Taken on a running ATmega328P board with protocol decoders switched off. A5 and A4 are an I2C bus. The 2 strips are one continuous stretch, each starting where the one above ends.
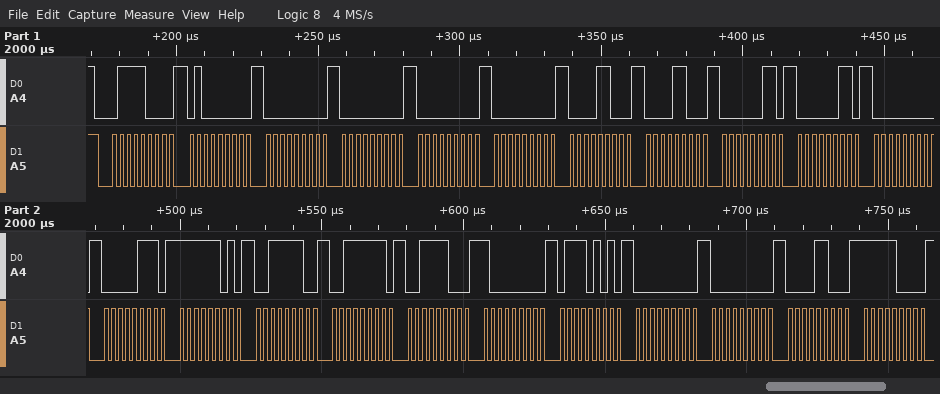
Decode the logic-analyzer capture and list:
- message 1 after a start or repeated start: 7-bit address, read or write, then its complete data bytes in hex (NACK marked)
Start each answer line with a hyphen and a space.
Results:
- 0x3C write: 40 00 00 00 00 0C 0C 03 03 00 07 FD 3E 3F 3C 80 75 00 00 0C F8
